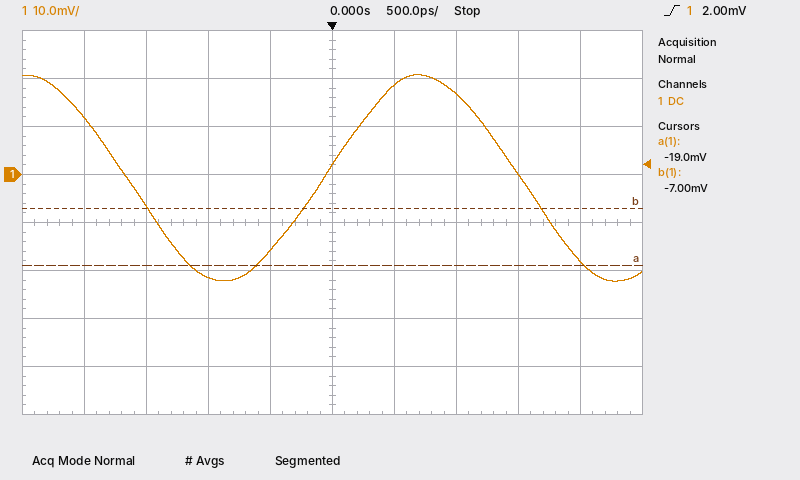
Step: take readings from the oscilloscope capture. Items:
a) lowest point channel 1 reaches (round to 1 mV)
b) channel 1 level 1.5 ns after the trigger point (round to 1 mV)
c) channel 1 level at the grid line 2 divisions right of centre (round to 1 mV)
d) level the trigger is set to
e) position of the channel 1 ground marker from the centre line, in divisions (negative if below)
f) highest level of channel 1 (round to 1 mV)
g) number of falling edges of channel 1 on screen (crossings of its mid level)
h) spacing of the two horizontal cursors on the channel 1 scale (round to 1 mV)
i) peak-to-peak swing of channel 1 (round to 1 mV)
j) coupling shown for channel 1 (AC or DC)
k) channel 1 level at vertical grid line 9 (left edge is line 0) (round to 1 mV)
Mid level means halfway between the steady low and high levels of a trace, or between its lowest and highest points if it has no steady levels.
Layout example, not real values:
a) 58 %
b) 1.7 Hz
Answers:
a) -22 mV
b) 0 mV
c) 17 mV
d) 2.00 mV
e) +1.0 div
f) 21 mV
g) 2
h) 12 mV
i) 43 mV
j) DC
k) -18 mV
